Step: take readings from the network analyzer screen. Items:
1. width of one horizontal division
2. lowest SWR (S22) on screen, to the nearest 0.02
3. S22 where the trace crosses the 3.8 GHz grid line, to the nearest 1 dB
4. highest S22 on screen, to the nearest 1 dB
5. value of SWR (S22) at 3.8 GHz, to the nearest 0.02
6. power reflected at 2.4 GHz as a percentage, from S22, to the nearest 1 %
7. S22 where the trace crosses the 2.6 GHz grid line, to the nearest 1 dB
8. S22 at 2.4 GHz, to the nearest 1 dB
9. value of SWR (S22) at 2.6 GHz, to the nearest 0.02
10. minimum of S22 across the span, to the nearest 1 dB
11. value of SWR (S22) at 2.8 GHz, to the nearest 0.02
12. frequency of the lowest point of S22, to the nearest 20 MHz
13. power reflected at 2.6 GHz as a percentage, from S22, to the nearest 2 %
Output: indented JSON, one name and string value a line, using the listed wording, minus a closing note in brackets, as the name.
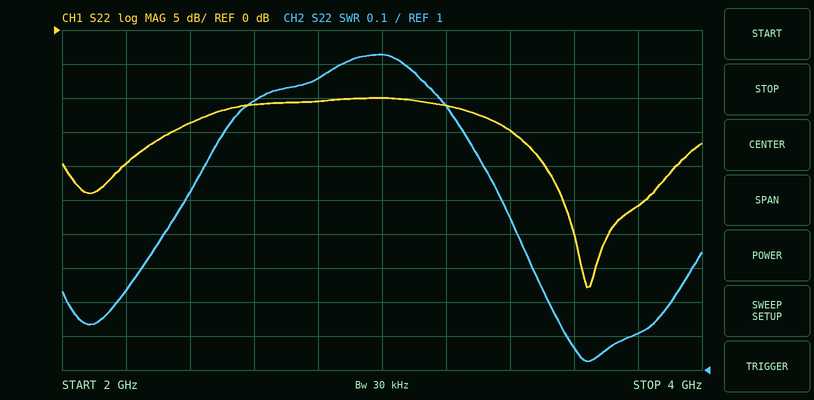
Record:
{
  "width of one horizontal division": "200 MHz",
  "lowest SWR (S22) on screen, to the nearest 0.02": "1.02",
  "S22 where the trace crosses the 3.8 GHz grid line, to the nearest 1 dB": "-26 dB",
  "highest S22 on screen, to the nearest 1 dB": "-10 dB",
  "value of SWR (S22) at 3.8 GHz, to the nearest 0.02": "1.10",
  "power reflected at 2.4 GHz as a percentage, from S22, to the nearest 1 %": "4 %",
  "S22 where the trace crosses the 2.6 GHz grid line, to the nearest 1 dB": "-11 dB",
  "S22 at 2.4 GHz, to the nearest 1 dB": "-14 dB",
  "value of SWR (S22) at 2.6 GHz, to the nearest 0.02": "1.80",
  "minimum of S22 across the span, to the nearest 1 dB": "-38 dB",
  "value of SWR (S22) at 2.8 GHz, to the nearest 0.02": "1.86",
  "frequency of the lowest point of S22, to the nearest 20 MHz": "3.64 GHz",
  "power reflected at 2.6 GHz as a percentage, from S22, to the nearest 2 %": "8 %"
}
